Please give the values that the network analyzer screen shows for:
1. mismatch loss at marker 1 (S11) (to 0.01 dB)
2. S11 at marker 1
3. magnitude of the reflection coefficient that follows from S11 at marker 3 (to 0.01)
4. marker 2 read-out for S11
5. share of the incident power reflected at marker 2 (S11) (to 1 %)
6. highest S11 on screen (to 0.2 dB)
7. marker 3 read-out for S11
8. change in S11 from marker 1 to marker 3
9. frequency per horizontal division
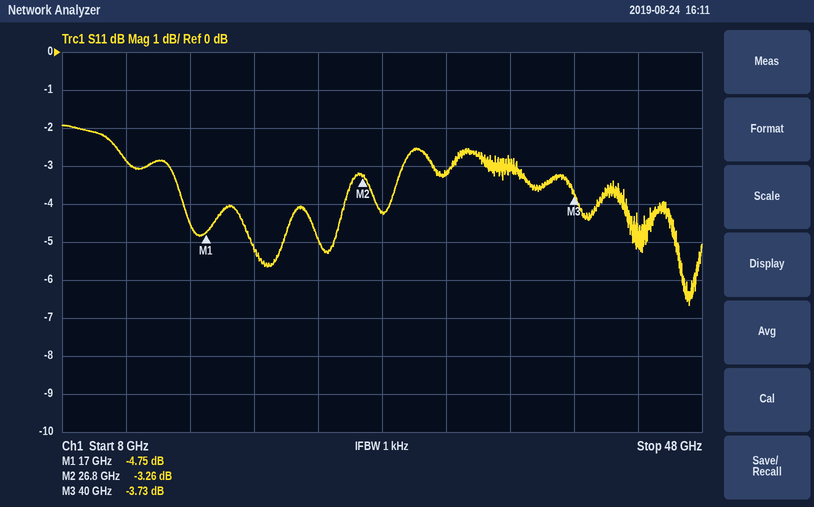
1.77 dB
-4.75 dB
0.65
-3.26 dB
47 %
-2.0 dB
-3.73 dB
1.02 dB
4 GHz
